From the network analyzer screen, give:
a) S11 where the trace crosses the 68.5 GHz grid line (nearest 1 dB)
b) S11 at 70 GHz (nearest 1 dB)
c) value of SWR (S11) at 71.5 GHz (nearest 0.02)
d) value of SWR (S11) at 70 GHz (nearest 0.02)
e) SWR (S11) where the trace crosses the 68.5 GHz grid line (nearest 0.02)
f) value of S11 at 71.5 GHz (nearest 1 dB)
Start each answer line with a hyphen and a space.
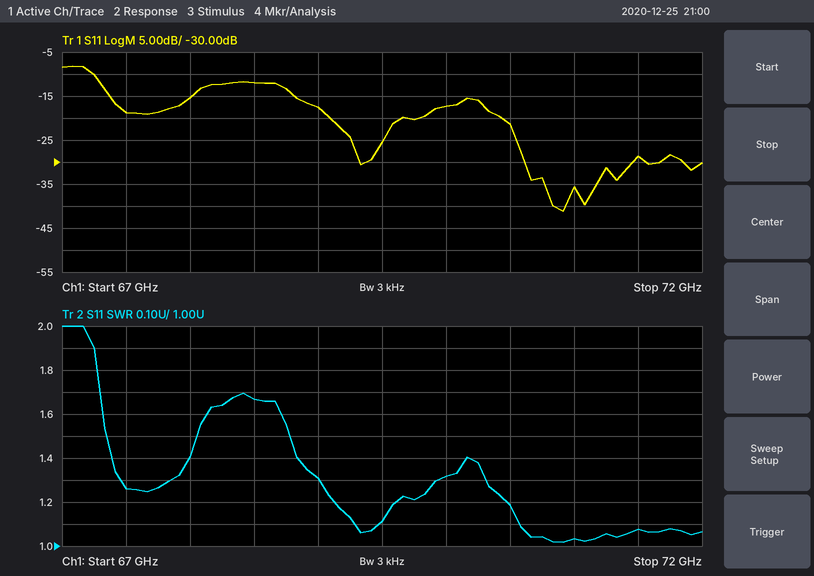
- -12 dB
- -17 dB
- 1.08
- 1.32
- 1.66
- -29 dB
